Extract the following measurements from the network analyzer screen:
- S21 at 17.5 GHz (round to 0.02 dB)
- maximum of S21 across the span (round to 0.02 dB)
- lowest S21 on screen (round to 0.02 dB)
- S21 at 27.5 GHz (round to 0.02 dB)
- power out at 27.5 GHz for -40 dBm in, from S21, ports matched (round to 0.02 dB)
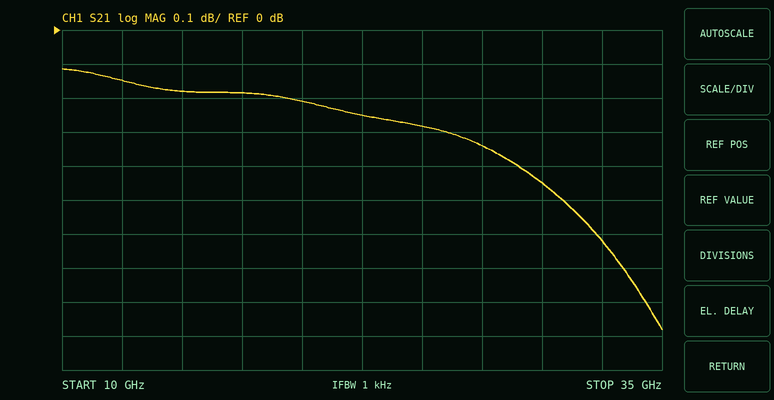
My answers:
-0.18 dB
-0.12 dB
-0.88 dB
-0.34 dB
-40.34 dBm
